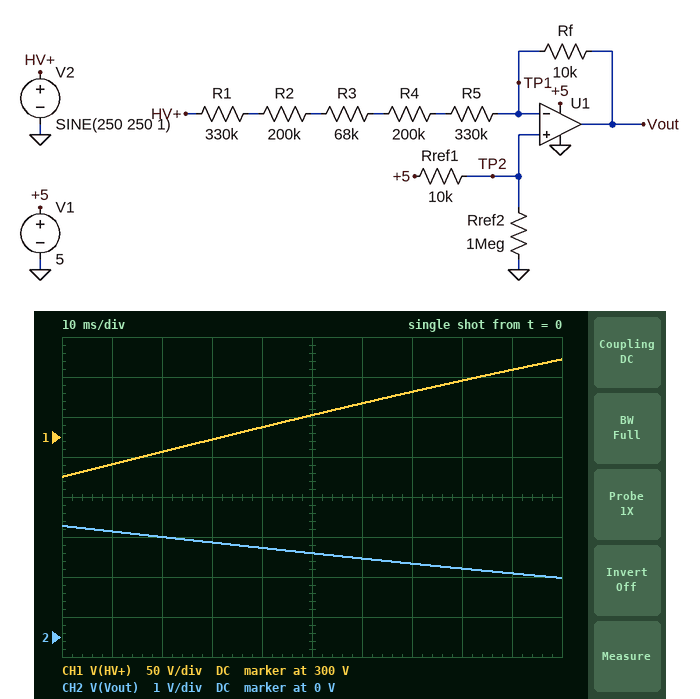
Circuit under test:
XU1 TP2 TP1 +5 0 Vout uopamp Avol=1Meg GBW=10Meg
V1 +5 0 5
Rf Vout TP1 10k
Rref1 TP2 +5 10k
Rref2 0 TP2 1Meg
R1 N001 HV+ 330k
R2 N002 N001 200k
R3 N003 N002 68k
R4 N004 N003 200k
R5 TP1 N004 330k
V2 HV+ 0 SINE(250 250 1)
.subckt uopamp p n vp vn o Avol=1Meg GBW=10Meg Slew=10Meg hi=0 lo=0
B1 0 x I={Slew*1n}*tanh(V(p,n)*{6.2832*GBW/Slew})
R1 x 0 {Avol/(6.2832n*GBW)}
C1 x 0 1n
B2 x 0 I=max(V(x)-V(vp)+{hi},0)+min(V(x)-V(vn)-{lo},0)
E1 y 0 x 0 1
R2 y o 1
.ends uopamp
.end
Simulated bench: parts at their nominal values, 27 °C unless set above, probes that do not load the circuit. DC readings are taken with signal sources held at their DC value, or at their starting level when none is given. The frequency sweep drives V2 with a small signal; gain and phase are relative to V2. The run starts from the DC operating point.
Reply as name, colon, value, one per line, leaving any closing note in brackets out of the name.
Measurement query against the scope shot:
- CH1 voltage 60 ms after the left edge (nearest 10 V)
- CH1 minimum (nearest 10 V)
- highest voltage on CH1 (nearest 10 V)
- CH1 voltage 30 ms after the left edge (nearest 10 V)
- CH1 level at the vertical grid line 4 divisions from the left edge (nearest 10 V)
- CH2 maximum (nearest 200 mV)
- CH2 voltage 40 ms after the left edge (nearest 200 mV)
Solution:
CH1 voltage 60 ms after the left edge: 340 V
CH1 minimum: 250 V
highest voltage on CH1: 400 V
CH1 voltage 30 ms after the left edge: 300 V
CH1 level at the vertical grid line 4 divisions from the left edge: 310 V
CH2 maximum: 2.8 V
CH2 voltage 40 ms after the left edge: 2.2 V
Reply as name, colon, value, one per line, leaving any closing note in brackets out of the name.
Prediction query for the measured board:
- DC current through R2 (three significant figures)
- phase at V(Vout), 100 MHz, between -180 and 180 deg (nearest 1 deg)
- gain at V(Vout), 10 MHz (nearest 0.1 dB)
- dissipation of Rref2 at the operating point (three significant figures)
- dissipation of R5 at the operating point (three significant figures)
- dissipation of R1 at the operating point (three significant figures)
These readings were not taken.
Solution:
DC current through R2: 217 µA
phase at V(Vout), 100 MHz, between -180 and 180 deg: 96 deg
gain at V(Vout), 10 MHz: -44.1 dB
dissipation of Rref2 at the operating point: 24.5 µW
dissipation of R5 at the operating point: 15.6 mW
dissipation of R1 at the operating point: 15.6 mW
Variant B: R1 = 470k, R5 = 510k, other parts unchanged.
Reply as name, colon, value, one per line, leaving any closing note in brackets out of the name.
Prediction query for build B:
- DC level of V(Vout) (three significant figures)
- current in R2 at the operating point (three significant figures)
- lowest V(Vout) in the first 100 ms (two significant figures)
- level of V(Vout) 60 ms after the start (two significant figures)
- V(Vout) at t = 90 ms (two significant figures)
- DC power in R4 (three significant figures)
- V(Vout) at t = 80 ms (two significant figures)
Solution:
DC level of V(Vout): 3.26 V
current in R2 at the operating point: 169 µA
lowest V(Vout) in the first 100 ms: 2.2 V
level of V(Vout) 60 ms after the start: 2.6 V
V(Vout) at t = 90 ms: 2.3 V
DC power in R4: 5.73 mW
V(Vout) at t = 80 ms: 2.4 V
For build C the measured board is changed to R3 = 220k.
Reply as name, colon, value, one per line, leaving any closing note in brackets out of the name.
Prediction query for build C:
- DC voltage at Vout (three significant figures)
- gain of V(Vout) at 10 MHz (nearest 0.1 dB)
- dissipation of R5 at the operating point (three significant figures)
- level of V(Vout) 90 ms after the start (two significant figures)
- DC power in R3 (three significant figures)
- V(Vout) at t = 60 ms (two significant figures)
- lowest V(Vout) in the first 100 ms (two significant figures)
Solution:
DC voltage at Vout: 3.04 V
gain of V(Vout) at 10 MHz: -45.2 dB
dissipation of R5 at the operating point: 12.1 mW
level of V(Vout) 90 ms after the start: 2.0 V
DC power in R3: 8.06 mW
V(Vout) at t = 60 ms: 2.3 V
lowest V(Vout) in the first 100 ms: 1.9 V
